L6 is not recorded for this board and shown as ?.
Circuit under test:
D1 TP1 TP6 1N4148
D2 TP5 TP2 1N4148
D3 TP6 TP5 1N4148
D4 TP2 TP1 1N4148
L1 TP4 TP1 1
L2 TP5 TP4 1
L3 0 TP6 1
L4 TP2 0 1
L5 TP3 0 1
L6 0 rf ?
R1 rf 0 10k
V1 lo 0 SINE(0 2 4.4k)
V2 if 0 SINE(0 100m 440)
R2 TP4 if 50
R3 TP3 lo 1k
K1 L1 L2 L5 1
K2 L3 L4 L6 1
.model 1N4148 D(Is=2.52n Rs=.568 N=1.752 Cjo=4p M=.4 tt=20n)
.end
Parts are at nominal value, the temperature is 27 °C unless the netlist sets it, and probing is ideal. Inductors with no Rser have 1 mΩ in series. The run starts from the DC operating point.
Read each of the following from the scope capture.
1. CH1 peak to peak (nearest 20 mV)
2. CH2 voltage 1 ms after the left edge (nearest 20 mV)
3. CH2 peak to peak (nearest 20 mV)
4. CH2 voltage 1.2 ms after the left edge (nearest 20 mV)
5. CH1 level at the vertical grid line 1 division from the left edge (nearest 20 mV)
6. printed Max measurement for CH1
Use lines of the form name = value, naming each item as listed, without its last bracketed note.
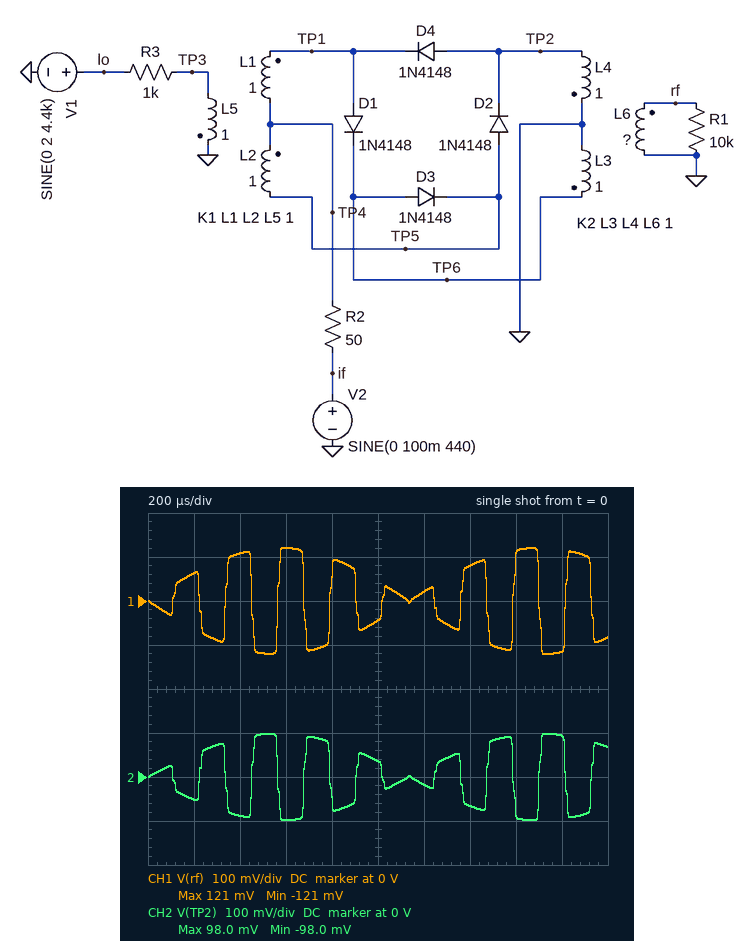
CH1 peak to peak = 240 mV
CH2 voltage 1 ms after the left edge = 40 mV
CH2 peak to peak = 200 mV
CH2 voltage 1.2 ms after the left edge = -20 mV
CH1 level at the vertical grid line 1 division from the left edge = 60 mV
printed Max measurement for CH1 = 121 mV
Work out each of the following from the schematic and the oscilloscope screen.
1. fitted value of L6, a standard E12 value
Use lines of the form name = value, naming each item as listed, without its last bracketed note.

fitted value of L6, a standard E12 value = 1.5 H
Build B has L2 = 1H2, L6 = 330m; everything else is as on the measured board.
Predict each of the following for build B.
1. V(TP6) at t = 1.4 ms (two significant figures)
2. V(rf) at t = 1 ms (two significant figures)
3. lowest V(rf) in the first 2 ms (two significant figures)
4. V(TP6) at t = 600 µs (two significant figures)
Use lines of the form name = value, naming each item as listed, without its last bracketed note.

V(TP6) at t = 1.4 ms = 42 mV
V(rf) at t = 1 ms = -34 mV
lowest V(rf) in the first 2 ms = -71 mV
V(TP6) at t = 600 µs = 75 mV
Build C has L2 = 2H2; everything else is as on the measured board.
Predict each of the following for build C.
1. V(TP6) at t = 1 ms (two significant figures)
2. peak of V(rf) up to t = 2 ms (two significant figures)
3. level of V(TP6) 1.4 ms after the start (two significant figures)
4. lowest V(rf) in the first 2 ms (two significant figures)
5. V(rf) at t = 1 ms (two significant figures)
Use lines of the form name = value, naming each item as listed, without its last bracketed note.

V(TP6) at t = 1 ms = -130 mV
peak of V(rf) up to t = 2 ms = 510 mV
level of V(TP6) 1.4 ms after the start = -32 mV
lowest V(rf) in the first 2 ms = -250 mV
V(rf) at t = 1 ms = -160 mV
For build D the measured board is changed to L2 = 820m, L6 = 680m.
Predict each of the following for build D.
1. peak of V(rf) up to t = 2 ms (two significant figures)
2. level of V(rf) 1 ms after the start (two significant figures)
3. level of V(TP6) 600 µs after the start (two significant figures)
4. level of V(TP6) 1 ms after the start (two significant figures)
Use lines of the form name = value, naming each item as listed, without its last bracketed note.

peak of V(rf) up to t = 2 ms = 100 mV
level of V(rf) 1 ms after the start = -9.9 mV
level of V(TP6) 600 µs after the start = 130 mV
level of V(TP6) 1 ms after the start = -12 mV
